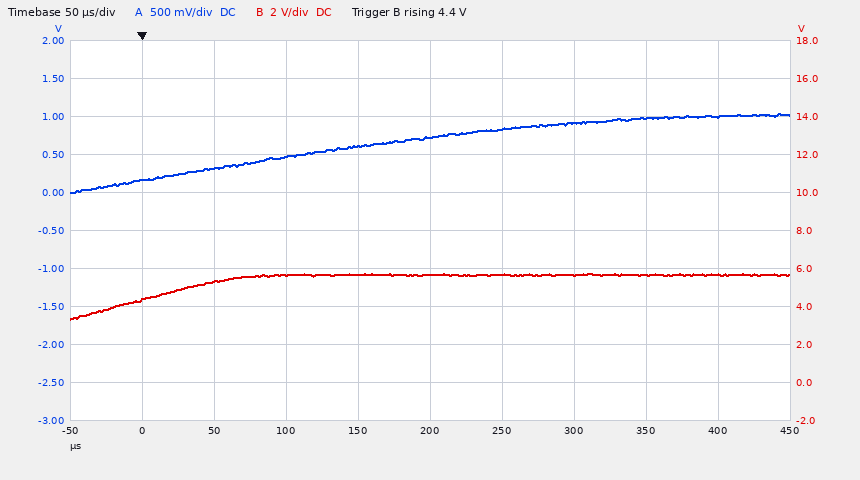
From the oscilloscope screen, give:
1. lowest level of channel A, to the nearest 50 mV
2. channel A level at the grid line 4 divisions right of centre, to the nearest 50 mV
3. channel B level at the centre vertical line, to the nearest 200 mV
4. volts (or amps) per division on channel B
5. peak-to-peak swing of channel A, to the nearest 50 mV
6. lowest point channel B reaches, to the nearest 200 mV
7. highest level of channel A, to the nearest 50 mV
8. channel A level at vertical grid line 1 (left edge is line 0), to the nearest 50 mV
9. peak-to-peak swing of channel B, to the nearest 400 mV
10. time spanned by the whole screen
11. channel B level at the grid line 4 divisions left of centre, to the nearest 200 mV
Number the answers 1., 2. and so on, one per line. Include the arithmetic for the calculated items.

1. 0 mV
2. 1.00 V
3. 5.6 V
4. 2 V
5. 1.05 V − (0 mV) = 1.05 V
6. 3.4 V
7. 1.05 V
8. 150 mV
9. 2.4 V
10. 500 µs
11. 4.4 V
